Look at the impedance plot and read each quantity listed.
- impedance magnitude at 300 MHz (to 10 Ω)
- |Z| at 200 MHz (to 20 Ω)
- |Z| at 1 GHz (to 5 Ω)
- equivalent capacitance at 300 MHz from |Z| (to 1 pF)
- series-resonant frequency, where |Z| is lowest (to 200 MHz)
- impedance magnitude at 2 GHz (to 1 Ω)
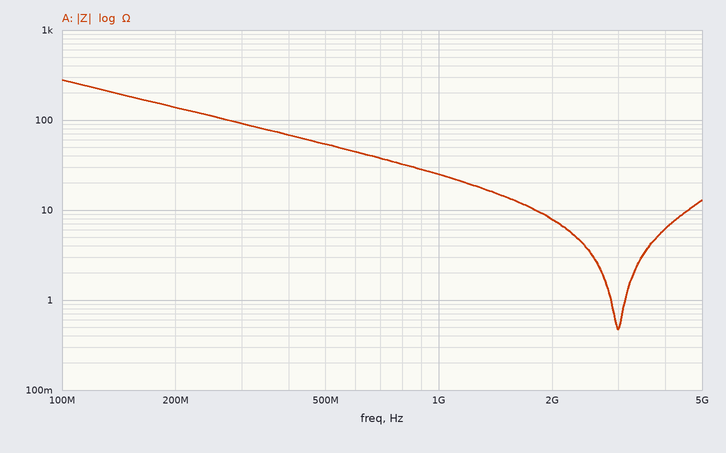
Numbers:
90 Ω
140 Ω
25 Ω
6 pF
3.0 GHz
8 Ω
